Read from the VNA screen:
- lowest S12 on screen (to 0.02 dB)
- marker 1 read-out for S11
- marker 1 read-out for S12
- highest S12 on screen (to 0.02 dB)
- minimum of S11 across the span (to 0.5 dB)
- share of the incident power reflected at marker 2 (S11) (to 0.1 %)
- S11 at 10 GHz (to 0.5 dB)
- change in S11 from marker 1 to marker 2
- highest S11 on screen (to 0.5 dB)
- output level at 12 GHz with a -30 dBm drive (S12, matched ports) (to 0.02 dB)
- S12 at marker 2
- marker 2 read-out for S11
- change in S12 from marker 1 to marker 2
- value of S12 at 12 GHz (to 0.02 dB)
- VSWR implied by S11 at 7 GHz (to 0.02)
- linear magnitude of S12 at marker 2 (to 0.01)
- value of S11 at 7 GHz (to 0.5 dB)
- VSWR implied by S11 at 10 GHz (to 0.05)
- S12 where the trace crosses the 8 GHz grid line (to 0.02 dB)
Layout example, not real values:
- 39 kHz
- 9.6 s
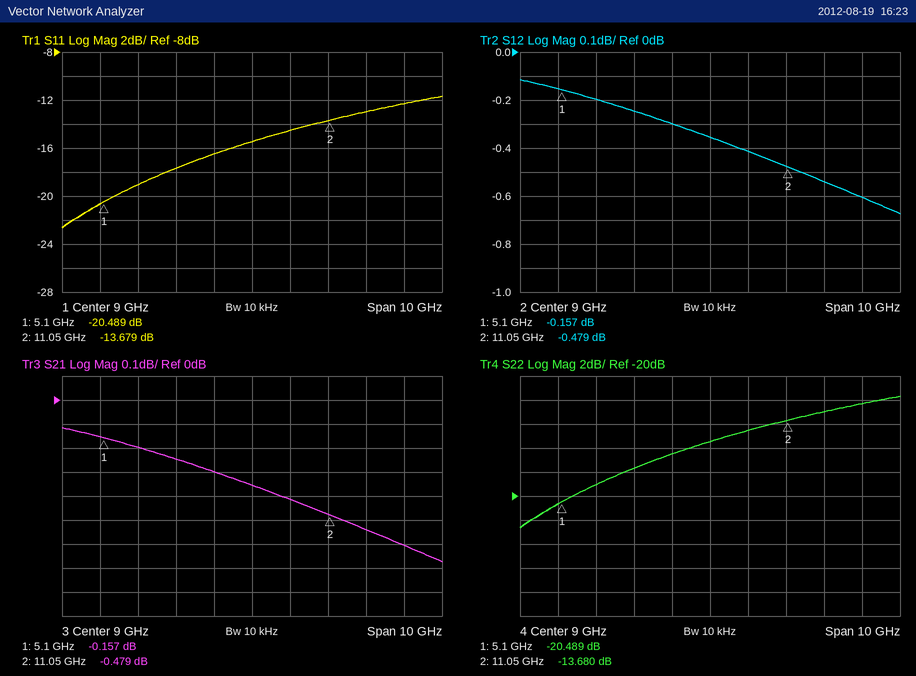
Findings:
- -0.68 dB
- -20.489 dB
- -0.157 dB
- -0.12 dB
- -22.5 dB
- 4.3 %
- -14.5 dB
- 6.810 dB
- -11.5 dB
- -30.54 dBm
- -0.479 dB
- -13.679 dB
- -0.322 dB
- -0.54 dB
- 1.30
- 0.95
- -17.5 dB
- 1.45
- -0.30 dB
